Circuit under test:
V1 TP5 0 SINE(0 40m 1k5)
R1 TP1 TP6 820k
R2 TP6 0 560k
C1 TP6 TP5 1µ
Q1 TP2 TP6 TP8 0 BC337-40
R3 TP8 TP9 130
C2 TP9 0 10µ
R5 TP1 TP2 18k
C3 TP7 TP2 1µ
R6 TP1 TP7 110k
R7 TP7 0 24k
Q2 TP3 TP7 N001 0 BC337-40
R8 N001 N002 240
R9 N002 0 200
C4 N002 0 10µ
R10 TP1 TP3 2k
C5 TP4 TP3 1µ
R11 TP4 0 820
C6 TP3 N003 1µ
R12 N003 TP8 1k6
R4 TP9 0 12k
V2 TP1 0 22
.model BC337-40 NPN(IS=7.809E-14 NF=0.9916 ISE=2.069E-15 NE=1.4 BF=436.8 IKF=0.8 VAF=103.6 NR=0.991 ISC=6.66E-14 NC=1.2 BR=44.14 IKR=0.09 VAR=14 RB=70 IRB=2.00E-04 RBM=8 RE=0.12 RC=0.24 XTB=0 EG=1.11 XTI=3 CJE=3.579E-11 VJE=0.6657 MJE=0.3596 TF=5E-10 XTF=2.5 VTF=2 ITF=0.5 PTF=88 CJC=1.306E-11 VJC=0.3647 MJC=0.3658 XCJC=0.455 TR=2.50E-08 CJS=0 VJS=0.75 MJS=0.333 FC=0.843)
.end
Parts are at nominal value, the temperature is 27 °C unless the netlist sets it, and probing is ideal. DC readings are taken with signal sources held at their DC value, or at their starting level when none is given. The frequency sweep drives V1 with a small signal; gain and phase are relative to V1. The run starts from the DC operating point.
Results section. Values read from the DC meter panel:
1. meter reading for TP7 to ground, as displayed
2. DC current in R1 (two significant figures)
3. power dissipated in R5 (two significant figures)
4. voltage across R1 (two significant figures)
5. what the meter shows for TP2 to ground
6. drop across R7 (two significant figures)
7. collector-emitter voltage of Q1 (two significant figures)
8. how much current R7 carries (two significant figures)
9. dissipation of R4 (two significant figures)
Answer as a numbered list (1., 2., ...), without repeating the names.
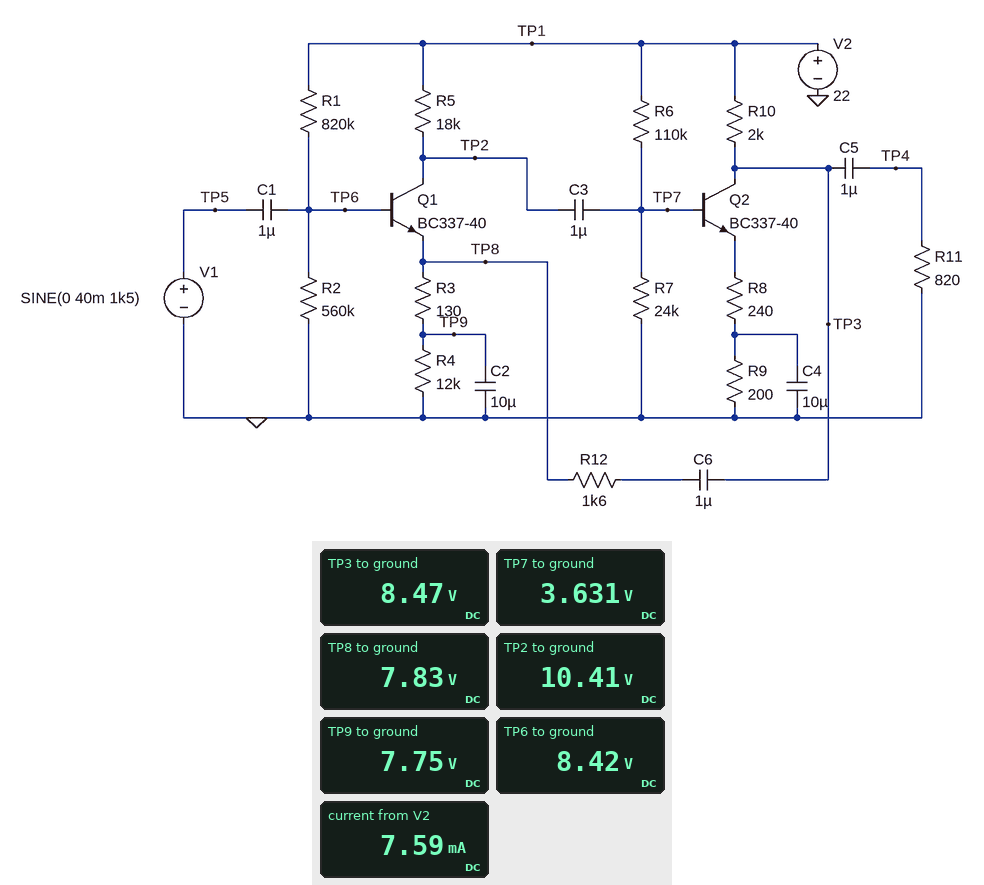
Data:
1. 3.631 V
2. 17 µA
3. 7.5 mW
4. 14 V
5. 10.41 V
6. 3.6 V
7. 2.6 V
8. 150 µA
9. 5.0 mW
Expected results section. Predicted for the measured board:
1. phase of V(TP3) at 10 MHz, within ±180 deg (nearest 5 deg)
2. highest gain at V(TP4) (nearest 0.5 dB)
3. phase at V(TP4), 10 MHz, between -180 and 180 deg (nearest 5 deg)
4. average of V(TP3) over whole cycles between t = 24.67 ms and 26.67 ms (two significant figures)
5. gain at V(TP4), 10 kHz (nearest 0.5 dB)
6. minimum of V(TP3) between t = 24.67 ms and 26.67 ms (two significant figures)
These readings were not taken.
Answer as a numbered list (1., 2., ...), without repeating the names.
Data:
1. -85 deg
2. 21.5 dB
3. -85 deg
4. 8.5 V
5. 21.5 dB
6. 8.0 V
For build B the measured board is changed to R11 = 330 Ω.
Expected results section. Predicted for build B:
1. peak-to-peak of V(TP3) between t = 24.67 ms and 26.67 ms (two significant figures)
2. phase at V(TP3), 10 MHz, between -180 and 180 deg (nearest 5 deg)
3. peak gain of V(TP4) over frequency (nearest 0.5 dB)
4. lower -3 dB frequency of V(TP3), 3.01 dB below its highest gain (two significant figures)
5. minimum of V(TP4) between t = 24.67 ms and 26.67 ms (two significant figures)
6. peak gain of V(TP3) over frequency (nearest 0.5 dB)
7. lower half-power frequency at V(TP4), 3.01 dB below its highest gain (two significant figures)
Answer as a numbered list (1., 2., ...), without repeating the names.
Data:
1. 860 mV
2. -95 deg
3. 20.5 dB
4. 3.4 Hz
5. -410 mV
6. 21.0 dB
7. 440 Hz
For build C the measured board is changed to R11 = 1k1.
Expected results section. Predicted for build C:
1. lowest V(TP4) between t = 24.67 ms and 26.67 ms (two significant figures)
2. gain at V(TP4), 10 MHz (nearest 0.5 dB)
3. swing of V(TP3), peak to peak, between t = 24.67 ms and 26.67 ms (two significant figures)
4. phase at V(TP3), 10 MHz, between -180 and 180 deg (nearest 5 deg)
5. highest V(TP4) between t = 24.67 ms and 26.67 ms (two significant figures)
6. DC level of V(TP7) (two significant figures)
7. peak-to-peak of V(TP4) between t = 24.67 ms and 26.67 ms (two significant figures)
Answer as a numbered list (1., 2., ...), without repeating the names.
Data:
1. -470 mV
2. 18.0 dB
3. 950 mV
4. -80 deg
5. 470 mV
6. 3.6 V
7. 940 mV
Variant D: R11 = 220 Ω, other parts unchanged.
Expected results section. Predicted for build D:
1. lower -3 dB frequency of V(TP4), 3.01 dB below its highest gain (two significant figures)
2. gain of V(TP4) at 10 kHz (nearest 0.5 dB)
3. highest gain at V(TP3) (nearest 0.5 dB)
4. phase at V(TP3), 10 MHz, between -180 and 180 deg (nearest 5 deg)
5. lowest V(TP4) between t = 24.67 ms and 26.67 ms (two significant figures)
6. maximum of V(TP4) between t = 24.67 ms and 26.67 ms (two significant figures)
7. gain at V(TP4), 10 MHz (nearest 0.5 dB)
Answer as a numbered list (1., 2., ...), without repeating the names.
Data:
1. 610 Hz
2. 20.0 dB
3. 21.0 dB
4. -95 deg
5. -370 mV
6. 370 mV
7. 11.5 dB
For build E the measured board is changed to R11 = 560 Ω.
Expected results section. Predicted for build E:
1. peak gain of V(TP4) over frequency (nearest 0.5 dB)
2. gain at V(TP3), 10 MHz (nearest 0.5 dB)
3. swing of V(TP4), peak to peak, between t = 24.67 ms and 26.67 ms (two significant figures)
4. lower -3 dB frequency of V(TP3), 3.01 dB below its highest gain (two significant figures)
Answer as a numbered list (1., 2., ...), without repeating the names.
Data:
1. 21.0 dB
2. 16.0 dB
3. 890 mV
4. 3.4 Hz
